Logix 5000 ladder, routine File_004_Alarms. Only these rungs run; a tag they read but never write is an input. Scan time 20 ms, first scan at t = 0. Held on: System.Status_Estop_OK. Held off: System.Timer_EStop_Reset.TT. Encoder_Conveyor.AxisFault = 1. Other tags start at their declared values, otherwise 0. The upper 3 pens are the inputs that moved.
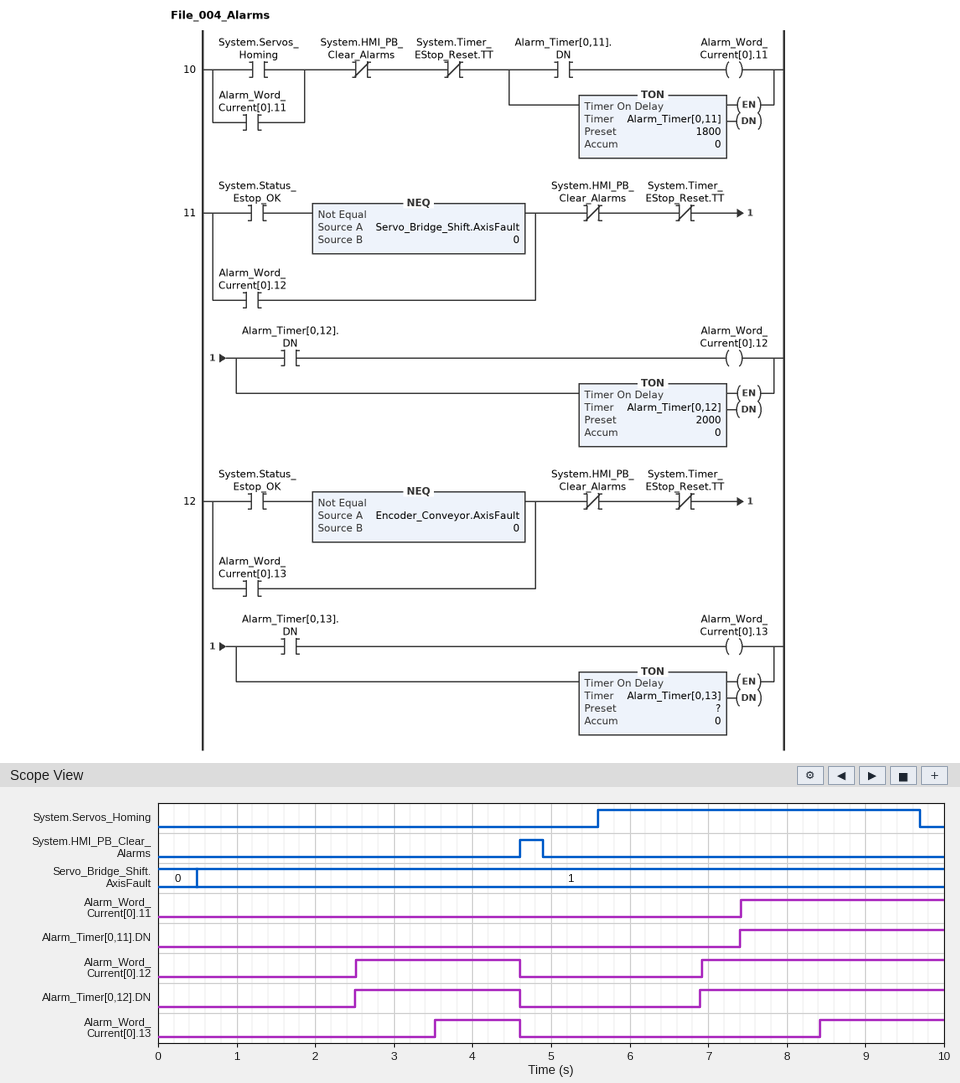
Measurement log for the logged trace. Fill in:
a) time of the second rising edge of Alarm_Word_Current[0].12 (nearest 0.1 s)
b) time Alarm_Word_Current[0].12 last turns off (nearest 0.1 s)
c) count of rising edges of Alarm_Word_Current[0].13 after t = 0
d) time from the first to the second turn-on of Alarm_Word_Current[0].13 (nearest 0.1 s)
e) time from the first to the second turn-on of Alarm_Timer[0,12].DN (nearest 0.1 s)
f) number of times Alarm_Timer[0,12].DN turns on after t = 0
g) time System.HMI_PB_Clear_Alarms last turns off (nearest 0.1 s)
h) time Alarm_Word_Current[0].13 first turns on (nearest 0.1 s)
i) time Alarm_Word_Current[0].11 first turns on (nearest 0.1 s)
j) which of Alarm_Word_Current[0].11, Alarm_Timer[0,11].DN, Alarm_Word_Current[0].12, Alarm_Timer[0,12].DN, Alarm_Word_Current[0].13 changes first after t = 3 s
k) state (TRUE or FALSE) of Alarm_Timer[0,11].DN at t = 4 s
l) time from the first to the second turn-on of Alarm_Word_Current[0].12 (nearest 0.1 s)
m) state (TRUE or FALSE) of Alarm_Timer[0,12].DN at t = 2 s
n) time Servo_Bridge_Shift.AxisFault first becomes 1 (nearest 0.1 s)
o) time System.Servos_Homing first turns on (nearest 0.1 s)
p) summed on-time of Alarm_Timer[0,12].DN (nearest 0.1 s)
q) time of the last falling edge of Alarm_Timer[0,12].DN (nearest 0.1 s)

6.9 s
4.6 s
2
4.9 s
4.4 s
2
4.9 s
3.5 s
7.4 s
Alarm_Word_Current[0].13
FALSE
4.4 s
FALSE
0.5 s
5.6 s
5.2 s
4.6 s
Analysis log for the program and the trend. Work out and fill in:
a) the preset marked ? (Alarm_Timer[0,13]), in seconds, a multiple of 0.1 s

3.5 s
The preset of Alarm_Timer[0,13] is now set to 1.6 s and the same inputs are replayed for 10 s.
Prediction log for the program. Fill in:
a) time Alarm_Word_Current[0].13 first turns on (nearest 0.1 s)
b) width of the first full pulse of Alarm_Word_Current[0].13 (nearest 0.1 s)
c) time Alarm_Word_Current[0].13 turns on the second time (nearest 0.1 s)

1.6 s
3.0 s
6.5 s
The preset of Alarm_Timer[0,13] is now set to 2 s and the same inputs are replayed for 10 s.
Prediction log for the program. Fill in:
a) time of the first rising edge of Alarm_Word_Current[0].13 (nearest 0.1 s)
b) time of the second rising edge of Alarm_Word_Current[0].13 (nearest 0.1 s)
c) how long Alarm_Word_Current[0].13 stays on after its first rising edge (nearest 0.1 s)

2.0 s
6.9 s
2.6 s
